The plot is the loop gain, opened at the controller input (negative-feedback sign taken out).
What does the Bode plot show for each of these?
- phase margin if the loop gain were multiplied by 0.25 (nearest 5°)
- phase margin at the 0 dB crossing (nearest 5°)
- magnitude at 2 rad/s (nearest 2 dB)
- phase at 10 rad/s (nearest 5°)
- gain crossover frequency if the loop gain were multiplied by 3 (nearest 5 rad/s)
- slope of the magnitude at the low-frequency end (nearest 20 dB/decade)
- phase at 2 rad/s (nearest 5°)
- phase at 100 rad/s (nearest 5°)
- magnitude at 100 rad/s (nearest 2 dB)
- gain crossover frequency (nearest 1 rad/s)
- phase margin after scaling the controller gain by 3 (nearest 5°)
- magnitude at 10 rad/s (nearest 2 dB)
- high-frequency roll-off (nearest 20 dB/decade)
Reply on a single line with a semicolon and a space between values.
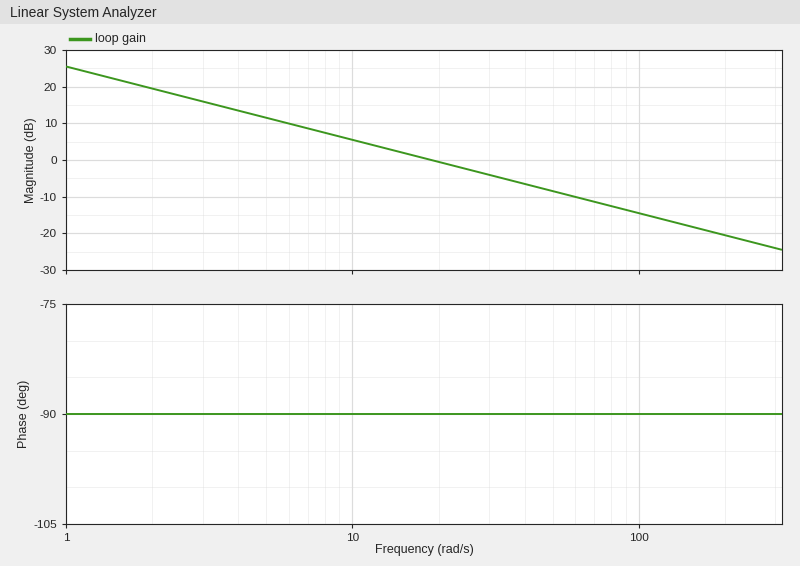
90°; 90°; 20 dB; -90°; 55 rad/s; -20 dB/decade; -90°; -90°; -14 dB; 19 rad/s; 90°; 6 dB; -20 dB/decade
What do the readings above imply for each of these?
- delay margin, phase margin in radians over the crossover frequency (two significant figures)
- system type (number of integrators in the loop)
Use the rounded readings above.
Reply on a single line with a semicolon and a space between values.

0.083 s; 1
